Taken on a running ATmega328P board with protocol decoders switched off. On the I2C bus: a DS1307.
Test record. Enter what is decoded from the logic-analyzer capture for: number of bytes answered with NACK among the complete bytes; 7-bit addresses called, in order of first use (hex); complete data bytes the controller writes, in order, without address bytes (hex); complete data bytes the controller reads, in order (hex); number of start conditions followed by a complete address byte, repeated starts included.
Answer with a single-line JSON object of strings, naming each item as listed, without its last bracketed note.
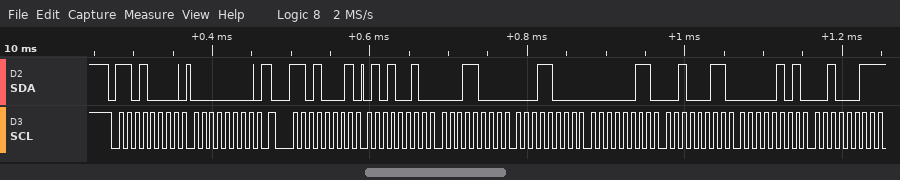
{"number of bytes answered with NACK among the complete bytes": "1", "7-bit addresses called, in order of first use": "0x68", "complete data bytes the controller writes, in order, without address bytes": "00", "complete data bytes the controller reads, in order": "52 18 18 03 23 05 23", "number of start conditions followed by a complete address byte, repeated starts included": "2"}
